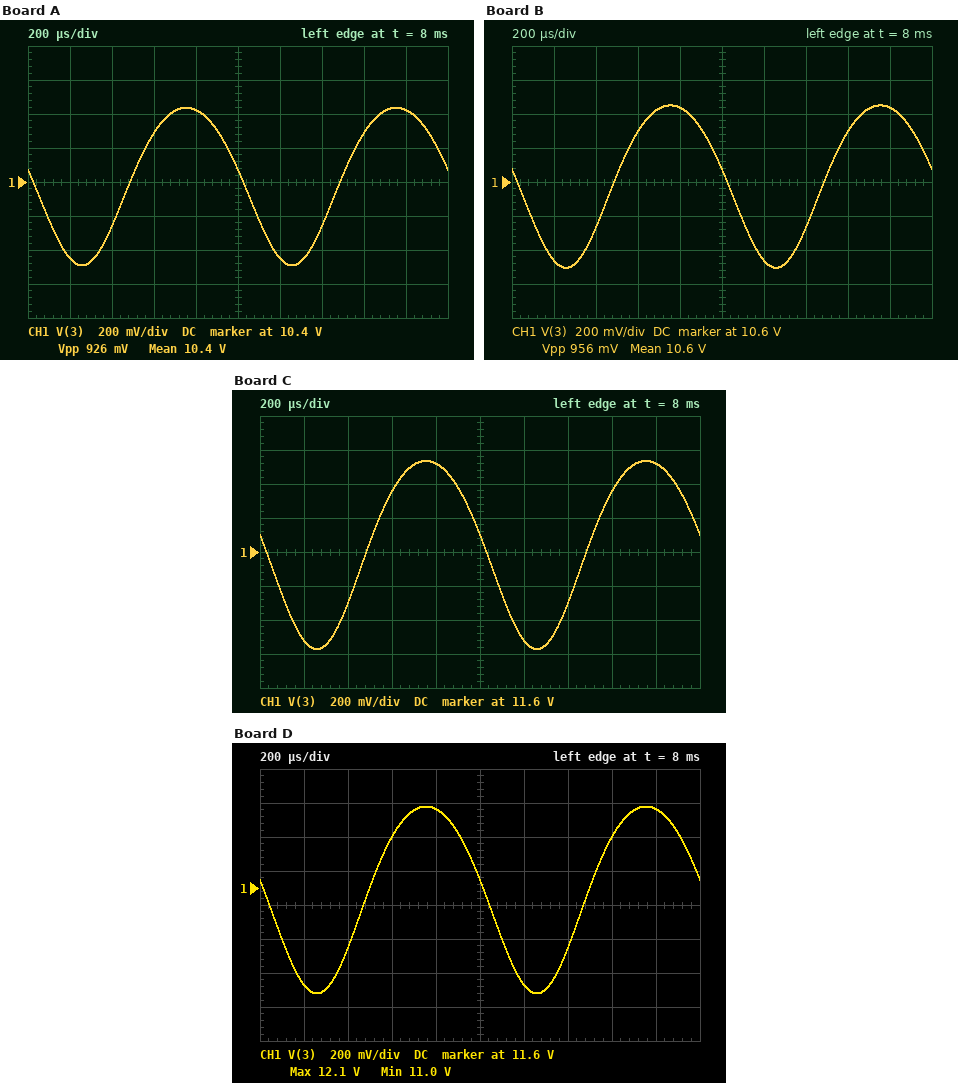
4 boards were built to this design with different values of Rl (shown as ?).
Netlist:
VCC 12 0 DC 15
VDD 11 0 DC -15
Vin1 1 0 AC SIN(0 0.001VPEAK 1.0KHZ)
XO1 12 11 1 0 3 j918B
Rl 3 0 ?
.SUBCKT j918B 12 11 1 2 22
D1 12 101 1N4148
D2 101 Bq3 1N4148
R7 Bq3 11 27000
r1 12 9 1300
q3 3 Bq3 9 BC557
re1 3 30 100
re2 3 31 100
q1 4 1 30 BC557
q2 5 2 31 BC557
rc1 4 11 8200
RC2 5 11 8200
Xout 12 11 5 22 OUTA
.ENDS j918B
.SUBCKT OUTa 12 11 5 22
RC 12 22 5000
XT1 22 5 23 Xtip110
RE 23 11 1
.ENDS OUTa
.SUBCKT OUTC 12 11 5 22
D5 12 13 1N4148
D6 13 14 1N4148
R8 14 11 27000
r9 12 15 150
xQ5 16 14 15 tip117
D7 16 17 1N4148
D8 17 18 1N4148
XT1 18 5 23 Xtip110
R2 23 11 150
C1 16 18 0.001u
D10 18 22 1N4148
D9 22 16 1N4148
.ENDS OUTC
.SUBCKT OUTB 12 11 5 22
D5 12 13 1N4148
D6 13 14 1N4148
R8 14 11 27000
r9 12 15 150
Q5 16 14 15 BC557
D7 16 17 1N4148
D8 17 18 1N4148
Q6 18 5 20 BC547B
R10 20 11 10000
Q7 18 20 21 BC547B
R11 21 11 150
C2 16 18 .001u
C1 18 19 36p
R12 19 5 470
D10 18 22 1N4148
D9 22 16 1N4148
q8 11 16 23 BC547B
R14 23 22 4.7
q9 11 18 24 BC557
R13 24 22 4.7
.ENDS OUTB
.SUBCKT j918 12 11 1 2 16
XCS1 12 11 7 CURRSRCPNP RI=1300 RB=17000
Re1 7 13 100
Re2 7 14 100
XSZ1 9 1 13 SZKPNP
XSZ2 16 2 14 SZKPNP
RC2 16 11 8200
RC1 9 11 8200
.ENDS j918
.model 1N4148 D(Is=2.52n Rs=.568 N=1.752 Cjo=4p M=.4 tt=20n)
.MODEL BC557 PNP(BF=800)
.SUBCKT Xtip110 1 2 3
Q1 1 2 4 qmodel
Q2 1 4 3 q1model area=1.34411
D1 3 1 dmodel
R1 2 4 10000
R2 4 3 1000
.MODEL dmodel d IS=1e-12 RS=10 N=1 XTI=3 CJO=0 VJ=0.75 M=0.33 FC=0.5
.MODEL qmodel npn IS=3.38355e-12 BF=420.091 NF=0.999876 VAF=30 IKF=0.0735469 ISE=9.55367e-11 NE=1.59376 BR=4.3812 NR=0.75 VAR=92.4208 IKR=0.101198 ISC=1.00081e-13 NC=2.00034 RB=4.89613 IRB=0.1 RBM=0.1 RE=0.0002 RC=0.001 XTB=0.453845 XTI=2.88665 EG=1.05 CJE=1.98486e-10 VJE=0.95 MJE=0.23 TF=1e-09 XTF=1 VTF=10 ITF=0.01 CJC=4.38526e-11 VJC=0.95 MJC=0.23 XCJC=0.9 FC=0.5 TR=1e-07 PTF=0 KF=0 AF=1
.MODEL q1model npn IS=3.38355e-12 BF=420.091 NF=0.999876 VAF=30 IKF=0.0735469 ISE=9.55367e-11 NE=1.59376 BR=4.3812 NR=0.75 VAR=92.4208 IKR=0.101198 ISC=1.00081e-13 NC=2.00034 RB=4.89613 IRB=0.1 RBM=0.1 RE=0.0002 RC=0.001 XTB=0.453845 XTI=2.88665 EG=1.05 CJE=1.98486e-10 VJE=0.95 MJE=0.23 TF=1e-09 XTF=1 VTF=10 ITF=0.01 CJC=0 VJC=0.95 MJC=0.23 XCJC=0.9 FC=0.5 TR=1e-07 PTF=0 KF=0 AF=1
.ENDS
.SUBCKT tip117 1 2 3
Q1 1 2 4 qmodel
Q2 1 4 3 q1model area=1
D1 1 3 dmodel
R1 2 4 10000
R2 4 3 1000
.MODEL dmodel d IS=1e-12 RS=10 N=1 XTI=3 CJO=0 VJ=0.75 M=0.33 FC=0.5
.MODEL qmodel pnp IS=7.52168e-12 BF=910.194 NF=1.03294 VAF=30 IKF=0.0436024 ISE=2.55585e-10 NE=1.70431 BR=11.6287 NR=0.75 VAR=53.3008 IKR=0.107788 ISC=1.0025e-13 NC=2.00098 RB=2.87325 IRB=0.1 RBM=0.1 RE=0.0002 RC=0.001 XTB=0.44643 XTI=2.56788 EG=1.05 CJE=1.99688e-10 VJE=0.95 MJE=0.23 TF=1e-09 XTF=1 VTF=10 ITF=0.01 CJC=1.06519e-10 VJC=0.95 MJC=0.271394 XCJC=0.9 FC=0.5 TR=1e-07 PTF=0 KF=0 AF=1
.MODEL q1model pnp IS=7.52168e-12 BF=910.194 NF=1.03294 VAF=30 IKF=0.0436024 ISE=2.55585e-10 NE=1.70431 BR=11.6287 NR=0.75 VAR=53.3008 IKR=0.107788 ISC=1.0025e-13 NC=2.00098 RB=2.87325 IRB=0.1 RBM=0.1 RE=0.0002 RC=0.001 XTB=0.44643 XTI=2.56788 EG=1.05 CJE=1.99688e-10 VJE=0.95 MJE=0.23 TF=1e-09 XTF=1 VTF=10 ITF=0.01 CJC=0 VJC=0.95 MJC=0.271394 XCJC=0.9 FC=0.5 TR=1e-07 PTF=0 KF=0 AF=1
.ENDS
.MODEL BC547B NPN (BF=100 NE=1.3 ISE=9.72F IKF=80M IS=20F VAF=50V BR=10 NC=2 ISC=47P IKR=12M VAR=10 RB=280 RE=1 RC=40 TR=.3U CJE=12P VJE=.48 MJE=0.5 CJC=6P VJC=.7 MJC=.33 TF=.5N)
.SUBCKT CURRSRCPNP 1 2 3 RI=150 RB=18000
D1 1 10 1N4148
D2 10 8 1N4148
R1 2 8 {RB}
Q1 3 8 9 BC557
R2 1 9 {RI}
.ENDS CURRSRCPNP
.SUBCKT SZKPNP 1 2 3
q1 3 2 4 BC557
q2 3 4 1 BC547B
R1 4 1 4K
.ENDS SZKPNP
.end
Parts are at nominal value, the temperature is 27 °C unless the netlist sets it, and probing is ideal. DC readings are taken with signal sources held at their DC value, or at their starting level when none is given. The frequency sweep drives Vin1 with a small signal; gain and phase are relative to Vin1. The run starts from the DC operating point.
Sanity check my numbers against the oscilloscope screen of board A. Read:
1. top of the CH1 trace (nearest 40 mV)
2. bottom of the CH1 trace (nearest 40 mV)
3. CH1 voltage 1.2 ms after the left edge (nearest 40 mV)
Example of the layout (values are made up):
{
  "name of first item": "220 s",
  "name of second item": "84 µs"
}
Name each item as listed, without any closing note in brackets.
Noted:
{
  "top of the CH1 trace": "10.84 V",
  "bottom of the CH1 trace": "9.92 V",
  "CH1 voltage 1.2 ms after the left edge": "9.96 V"
}
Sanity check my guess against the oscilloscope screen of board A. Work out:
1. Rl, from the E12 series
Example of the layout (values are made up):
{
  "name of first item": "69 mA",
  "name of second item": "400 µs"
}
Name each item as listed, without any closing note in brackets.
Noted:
{
  "Rl, from the E12 series": "33 kΩ"
}
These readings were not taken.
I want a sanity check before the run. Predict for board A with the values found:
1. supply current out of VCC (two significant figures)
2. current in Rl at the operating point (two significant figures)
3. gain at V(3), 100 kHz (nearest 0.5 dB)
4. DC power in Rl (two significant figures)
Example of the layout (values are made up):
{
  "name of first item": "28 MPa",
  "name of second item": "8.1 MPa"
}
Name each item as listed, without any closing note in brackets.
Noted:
{
  "supply current out of VCC": "2.3 mA",
  "current in Rl at the operating point": "320 µA",
  "gain at V(3), 100 kHz": "42.5 dB",
  "DC power in Rl": "3.3 mW"
}
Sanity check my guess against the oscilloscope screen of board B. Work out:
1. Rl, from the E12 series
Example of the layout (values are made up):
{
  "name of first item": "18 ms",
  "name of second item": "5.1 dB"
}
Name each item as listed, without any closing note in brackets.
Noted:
{
  "Rl, from the E12 series": "39 kΩ"
}
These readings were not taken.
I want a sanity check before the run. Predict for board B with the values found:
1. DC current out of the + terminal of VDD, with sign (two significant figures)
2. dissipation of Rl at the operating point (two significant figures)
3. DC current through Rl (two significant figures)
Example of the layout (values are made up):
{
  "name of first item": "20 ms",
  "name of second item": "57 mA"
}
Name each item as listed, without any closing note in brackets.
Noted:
{
  "DC current out of the + terminal of VDD, with sign": "-2.0 mA",
  "dissipation of Rl at the operating point": "2.9 mW",
  "DC current through Rl": "270 µA"
}
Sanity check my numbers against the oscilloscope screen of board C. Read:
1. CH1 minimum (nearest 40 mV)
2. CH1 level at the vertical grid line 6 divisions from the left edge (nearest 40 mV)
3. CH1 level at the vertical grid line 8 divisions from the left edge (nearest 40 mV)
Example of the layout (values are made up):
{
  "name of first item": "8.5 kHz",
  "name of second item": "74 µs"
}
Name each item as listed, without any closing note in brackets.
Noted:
{
  "CH1 minimum": "11.04 V",
  "CH1 level at the vertical grid line 6 divisions from the left edge": "11.08 V",
  "CH1 level at the vertical grid line 8 divisions from the left edge": "11.96 V"
}
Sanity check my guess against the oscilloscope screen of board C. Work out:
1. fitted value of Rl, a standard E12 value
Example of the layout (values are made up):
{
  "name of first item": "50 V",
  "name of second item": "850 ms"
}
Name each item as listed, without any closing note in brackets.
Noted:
{
  "fitted value of Rl, a standard E12 value": "220 kΩ"
}
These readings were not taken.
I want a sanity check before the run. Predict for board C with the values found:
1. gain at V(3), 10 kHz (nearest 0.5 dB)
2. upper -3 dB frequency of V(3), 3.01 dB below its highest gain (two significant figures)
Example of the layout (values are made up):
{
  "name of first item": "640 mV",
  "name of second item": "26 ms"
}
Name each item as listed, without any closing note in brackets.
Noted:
{
  "gain at V(3), 10 kHz": "54.0 dB",
  "upper -3 dB frequency of V(3), 3.01 dB below its highest gain": "26 kHz"
}
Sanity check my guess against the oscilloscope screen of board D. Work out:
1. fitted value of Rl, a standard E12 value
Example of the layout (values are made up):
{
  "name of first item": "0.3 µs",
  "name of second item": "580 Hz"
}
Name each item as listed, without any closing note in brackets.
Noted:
{
  "fitted value of Rl, a standard E12 value": "180 kΩ"
}
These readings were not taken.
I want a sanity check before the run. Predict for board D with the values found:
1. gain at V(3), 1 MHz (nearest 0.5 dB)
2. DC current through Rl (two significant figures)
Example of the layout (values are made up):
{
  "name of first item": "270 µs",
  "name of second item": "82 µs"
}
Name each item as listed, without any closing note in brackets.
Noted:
{
  "gain at V(3), 1 MHz": "23.0 dB",
  "DC current through Rl": "65 µA"
}
